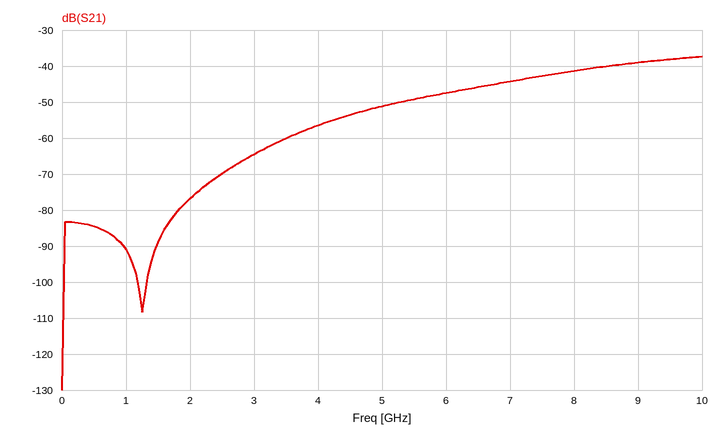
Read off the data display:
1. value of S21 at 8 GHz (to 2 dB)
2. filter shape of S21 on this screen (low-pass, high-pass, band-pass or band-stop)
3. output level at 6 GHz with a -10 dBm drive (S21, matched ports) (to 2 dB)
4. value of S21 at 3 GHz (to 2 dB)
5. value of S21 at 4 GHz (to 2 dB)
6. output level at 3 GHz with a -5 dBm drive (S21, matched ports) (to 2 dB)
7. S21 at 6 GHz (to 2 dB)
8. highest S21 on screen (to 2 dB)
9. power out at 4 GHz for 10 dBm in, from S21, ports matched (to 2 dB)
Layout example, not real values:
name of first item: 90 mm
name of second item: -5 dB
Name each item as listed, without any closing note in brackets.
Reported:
value of S21 at 8 GHz: -42 dB
filter shape of S21 on this screen: high-pass
output level at 6 GHz with a -10 dBm drive (S21, matched ports): -58 dBm
value of S21 at 3 GHz: -64 dB
value of S21 at 4 GHz: -56 dB
output level at 3 GHz with a -5 dBm drive (S21, matched ports): -70 dBm
S21 at 6 GHz: -48 dB
highest S21 on screen: -38 dB
power out at 4 GHz for 10 dBm in, from S21, ports matched: -46 dBm
